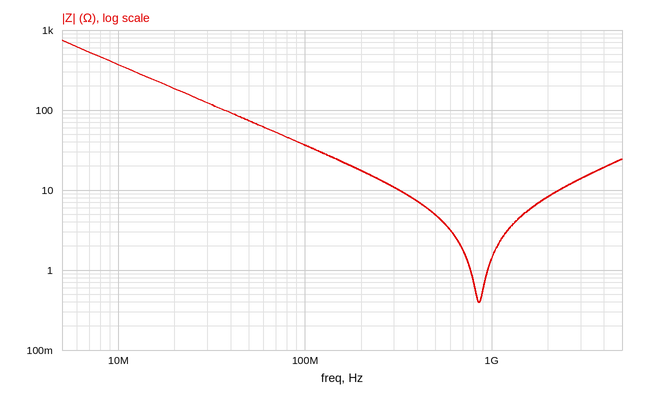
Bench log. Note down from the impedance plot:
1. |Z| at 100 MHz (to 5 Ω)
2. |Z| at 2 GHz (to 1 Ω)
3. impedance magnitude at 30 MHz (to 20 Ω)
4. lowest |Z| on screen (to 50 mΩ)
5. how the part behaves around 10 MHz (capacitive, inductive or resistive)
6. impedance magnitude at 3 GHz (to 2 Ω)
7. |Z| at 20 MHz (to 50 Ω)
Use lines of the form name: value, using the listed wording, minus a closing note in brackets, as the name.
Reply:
|Z| at 100 MHz: 35 Ω
|Z| at 2 GHz: 8 Ω
impedance magnitude at 30 MHz: 120 Ω
lowest |Z| on screen: 400 mΩ
how the part behaves around 10 MHz: capacitive
impedance magnitude at 3 GHz: 14 Ω
|Z| at 20 MHz: 200 Ω
